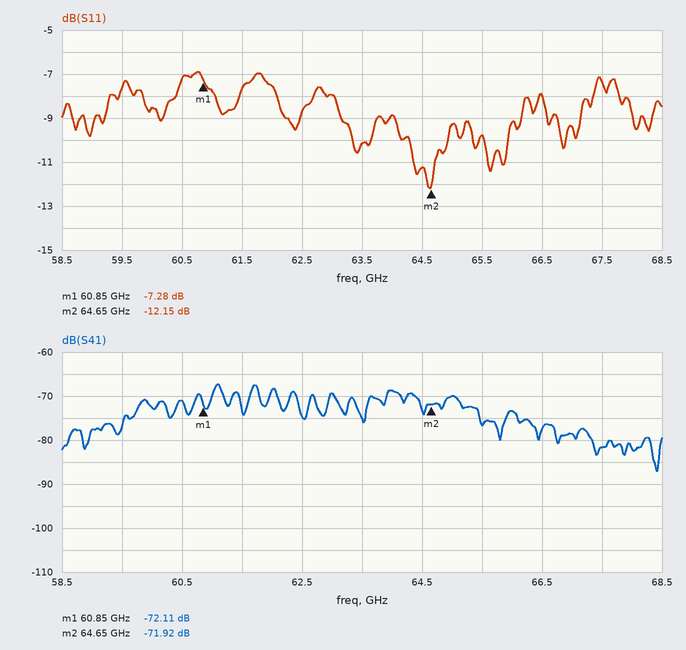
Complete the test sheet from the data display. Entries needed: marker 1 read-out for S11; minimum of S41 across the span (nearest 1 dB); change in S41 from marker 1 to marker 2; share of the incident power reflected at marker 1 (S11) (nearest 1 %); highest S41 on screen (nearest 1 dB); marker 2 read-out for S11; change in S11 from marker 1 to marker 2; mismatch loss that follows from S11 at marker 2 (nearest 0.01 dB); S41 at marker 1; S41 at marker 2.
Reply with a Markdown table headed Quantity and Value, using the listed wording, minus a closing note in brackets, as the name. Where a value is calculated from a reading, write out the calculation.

| Quantity | Value |
|---|---|
| marker 1 read-out for S11 | -7.28 dB |
| minimum of S41 across the span | -87 dB |
| change in S41 from marker 1 to marker 2 | -71.92 − (-72.11) = 0.19 dB |
| share of the incident power reflected at marker 1 (S11) | 10^(-7.28/10) ≈ 19 % |
| highest S41 on screen | -67 dB |
| marker 2 read-out for S11 | -12.15 dB |
| change in S11 from marker 1 to marker 2 | -12.15 − (-7.28) = -4.87 dB |
| mismatch loss that follows from S11 at marker 2 | −10 log10(1 − 10^(-12.15/10)) ≈ 0.27 dB |
| S41 at marker 1 | -72.11 dB |
| S41 at marker 2 | -71.92 dB |
